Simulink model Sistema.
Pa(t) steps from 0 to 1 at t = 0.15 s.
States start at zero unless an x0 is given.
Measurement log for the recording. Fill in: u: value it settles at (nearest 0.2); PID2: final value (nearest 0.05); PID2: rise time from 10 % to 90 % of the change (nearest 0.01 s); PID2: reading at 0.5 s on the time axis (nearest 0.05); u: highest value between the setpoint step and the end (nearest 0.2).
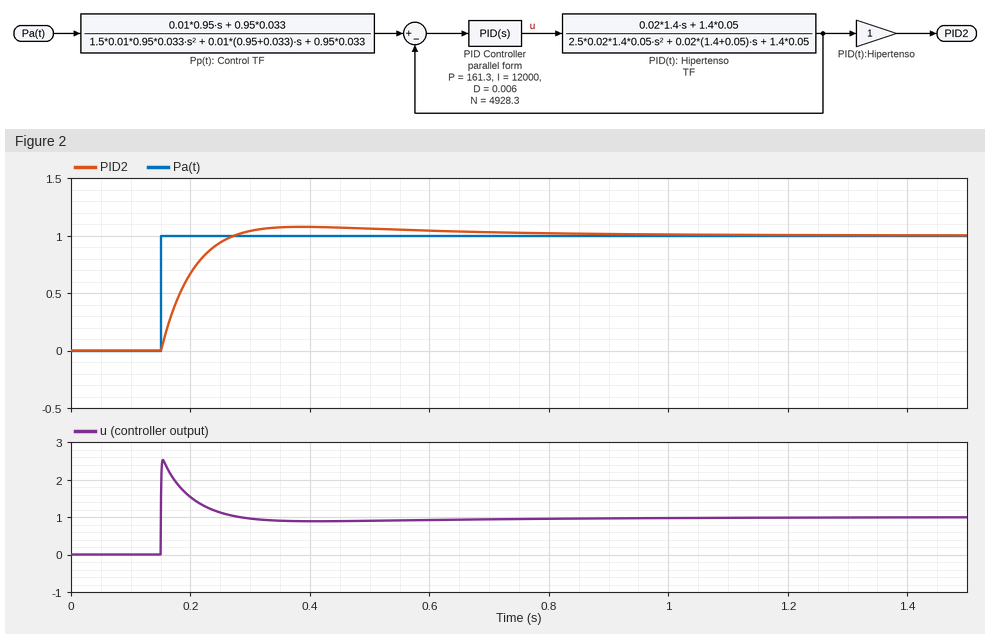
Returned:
1.0
1.00
0.08 s
1.05
2.6
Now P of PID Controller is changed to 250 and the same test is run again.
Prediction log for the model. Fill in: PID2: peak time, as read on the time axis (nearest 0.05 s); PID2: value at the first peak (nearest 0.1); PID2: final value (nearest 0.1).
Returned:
0.40 s
1.1
1.0
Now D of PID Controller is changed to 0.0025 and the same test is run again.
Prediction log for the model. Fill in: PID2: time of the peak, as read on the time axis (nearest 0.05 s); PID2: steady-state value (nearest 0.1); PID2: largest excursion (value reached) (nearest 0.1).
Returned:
0.40 s
1.0
1.1
